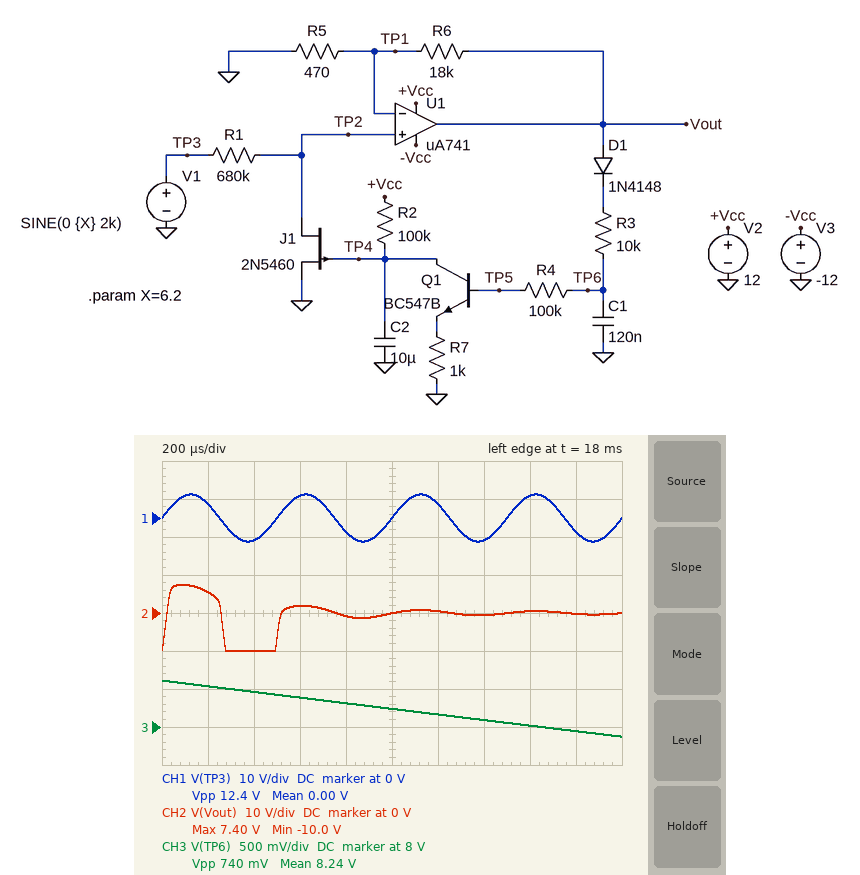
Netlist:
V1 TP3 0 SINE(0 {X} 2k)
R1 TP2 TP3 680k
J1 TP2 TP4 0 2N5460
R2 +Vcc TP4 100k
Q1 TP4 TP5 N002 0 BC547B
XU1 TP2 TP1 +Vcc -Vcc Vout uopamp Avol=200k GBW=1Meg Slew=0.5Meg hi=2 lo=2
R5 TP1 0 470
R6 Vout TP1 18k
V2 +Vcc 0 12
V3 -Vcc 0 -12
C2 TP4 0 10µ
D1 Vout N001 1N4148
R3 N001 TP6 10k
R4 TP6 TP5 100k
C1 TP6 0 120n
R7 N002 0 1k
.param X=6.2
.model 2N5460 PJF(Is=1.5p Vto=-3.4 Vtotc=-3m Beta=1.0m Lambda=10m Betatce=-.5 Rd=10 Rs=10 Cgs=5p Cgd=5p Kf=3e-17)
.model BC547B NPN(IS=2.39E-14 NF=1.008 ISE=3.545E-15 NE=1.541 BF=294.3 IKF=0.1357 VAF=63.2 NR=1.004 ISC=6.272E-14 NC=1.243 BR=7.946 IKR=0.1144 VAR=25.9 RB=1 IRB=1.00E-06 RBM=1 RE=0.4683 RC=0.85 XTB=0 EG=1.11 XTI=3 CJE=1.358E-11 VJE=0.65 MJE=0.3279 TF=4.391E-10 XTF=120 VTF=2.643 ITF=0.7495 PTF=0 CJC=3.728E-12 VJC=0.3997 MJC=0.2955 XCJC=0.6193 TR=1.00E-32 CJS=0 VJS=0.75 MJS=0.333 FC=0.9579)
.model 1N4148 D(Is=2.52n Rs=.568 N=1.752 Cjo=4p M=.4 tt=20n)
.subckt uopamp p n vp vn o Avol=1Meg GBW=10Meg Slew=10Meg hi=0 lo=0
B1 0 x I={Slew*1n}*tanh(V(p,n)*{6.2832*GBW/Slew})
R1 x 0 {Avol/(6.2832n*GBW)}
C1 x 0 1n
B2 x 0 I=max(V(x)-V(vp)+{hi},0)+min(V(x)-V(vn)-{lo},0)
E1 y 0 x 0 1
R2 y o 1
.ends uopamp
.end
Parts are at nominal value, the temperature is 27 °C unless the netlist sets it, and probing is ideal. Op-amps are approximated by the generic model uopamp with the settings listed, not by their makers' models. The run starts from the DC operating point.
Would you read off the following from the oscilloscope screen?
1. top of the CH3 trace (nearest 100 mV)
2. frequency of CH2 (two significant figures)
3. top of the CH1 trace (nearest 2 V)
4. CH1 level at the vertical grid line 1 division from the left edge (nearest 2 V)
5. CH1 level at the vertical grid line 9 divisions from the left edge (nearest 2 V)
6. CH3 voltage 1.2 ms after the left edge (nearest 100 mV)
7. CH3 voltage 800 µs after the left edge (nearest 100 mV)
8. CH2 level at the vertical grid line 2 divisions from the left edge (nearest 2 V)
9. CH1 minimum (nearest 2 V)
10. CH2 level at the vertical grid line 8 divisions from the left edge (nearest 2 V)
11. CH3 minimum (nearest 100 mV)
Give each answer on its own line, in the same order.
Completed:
8.6 V
2.0 kHz
6 V
4 V
-4 V
8.2 V
8.3 V
-10 V
-6 V
0 V
7.9 V
